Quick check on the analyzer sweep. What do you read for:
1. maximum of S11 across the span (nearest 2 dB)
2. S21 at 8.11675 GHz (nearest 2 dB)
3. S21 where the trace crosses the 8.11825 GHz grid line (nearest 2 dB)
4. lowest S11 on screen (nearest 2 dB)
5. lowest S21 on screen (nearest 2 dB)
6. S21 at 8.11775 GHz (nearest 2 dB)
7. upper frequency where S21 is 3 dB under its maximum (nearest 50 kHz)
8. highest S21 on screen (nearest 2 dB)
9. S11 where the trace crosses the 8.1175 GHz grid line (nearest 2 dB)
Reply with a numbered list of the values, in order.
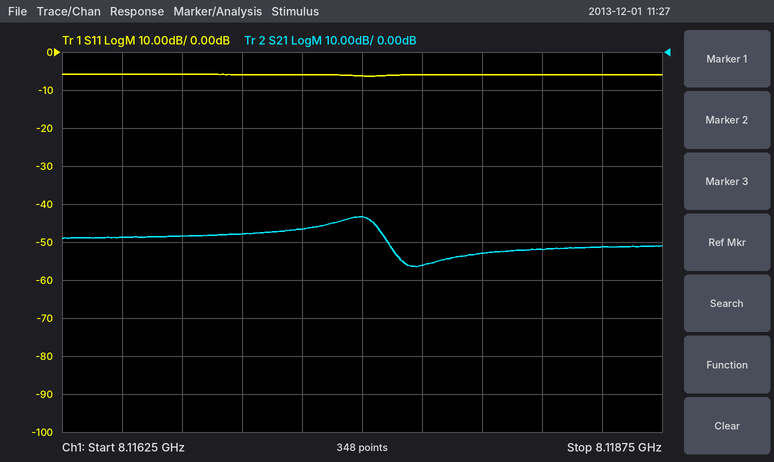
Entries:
1. -6 dB
2. -48 dB
3. -52 dB
4. -6 dB
5. -56 dB
6. -56 dB
7. 8.11755 GHz
8. -44 dB
9. -6 dB
